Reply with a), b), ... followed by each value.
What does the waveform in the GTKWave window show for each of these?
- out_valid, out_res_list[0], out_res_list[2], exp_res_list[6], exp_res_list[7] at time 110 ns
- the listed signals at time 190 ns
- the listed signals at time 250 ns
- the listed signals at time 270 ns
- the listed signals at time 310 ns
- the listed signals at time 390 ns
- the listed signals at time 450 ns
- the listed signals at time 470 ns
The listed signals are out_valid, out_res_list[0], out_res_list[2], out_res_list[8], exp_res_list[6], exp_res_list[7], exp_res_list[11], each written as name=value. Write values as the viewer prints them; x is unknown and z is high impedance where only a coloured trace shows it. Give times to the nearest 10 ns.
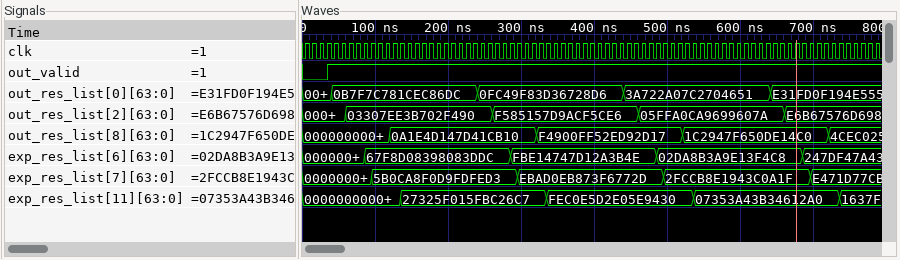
a) out_valid=1, out_res_list[0]=0B7F7C781CEC86DC, out_res_list[2]=03307EE3B702F490, exp_res_list[6]=67F8D08398083DDC, exp_res_list[7]=5B0CA8F0D9FDFED3
b) out_valid=1, out_res_list[0]=0B7F7C781CEC86DC, out_res_list[2]=03307EE3B702F490, out_res_list[8]=0A1E4D147D41CB10, exp_res_list[6]=67F8D08398083DDC, exp_res_list[7]=5B0CA8F0D9FDFED3, exp_res_list[11]=27325F015FBC26C7
c) out_valid=1, out_res_list[0]=0FC49F83D36728D6, out_res_list[2]=03307EE3B702F490, out_res_list[8]=0A1E4D147D41CB10, exp_res_list[6]=67F8D08398083DDC, exp_res_list[7]=5B0CA8F0D9FDFED3, exp_res_list[11]=27325F015FBC26C7
d) out_valid=1, out_res_list[0]=0FC49F83D36728D6, out_res_list[2]=F585157D9ACF5CE6, out_res_list[8]=0A1E4D147D41CB10, exp_res_list[6]=67F8D08398083DDC, exp_res_list[7]=5B0CA8F0D9FDFED3, exp_res_list[11]=27325F015FBC26C7
e) out_valid=1, out_res_list[0]=0FC49F83D36728D6, out_res_list[2]=F585157D9ACF5CE6, out_res_list[8]=0A1E4D147D41CB10, exp_res_list[6]=FBE14747D12A3B4E, exp_res_list[7]=EBAD0EB873F6772D, exp_res_list[11]=27325F015FBC26C7
f) out_valid=1, out_res_list[0]=0FC49F83D36728D6, out_res_list[2]=F585157D9ACF5CE6, out_res_list[8]=F4900FF52ED92D17, exp_res_list[6]=FBE14747D12A3B4E, exp_res_list[7]=EBAD0EB873F6772D, exp_res_list[11]=FEC0E5D2E05E9430
g) out_valid=1, out_res_list[0]=3A722A07C2704651, out_res_list[2]=F585157D9ACF5CE6, out_res_list[8]=F4900FF52ED92D17, exp_res_list[6]=FBE14747D12A3B4E, exp_res_list[7]=EBAD0EB873F6772D, exp_res_list[11]=FEC0E5D2E05E9430
h) out_valid=1, out_res_list[0]=3A722A07C2704651, out_res_list[2]=05FFA0CA9699607A, out_res_list[8]=F4900FF52ED92D17, exp_res_list[6]=FBE14747D12A3B4E, exp_res_list[7]=EBAD0EB873F6772D, exp_res_list[11]=FEC0E5D2E05E9430
